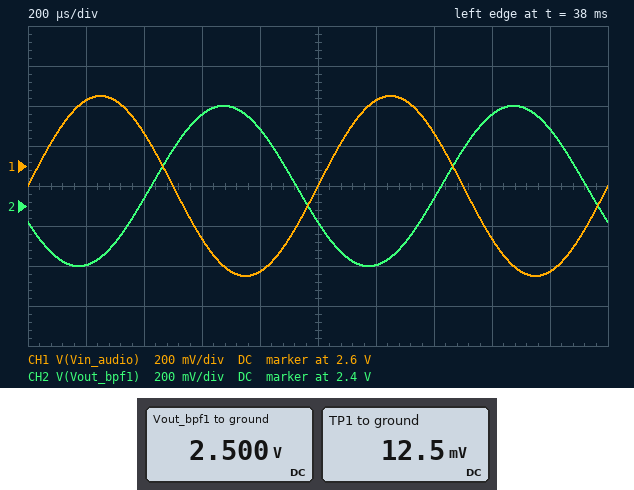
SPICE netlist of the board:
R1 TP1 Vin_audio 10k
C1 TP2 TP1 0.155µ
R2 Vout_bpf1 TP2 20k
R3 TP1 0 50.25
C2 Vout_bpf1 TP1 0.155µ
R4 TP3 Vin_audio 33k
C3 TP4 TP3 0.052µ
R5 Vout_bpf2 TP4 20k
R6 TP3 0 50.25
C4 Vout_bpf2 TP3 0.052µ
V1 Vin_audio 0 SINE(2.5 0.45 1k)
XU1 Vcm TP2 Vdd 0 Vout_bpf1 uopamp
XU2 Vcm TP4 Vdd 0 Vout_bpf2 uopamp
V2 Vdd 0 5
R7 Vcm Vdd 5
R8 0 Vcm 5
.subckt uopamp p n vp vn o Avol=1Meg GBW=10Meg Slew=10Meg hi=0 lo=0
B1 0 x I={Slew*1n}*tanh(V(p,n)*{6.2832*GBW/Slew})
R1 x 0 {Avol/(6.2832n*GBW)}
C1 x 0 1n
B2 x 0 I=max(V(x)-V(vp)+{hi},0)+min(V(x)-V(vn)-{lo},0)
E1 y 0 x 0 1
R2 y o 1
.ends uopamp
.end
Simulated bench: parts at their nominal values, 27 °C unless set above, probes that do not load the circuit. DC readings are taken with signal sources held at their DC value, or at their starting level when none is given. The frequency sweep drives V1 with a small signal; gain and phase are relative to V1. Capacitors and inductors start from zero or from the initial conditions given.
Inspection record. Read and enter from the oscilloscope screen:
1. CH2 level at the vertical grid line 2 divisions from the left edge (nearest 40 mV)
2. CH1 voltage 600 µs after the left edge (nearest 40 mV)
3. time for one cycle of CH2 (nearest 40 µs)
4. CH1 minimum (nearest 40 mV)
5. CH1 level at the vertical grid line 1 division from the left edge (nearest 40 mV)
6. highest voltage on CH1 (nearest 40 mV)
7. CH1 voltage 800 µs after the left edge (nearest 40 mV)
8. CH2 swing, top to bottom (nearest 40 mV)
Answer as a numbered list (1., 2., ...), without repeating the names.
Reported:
1. 2.44 V
2. 2.24 V
3. 1.00 ms
4. 2.04 V
5. 2.92 V
6. 2.96 V
7. 2.08 V
8. 800 mV
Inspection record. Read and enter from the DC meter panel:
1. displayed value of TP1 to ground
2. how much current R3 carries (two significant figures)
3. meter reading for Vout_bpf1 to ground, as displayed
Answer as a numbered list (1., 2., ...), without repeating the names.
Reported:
1. 12.5 mV
2. 250 µA
3. 2.500 V
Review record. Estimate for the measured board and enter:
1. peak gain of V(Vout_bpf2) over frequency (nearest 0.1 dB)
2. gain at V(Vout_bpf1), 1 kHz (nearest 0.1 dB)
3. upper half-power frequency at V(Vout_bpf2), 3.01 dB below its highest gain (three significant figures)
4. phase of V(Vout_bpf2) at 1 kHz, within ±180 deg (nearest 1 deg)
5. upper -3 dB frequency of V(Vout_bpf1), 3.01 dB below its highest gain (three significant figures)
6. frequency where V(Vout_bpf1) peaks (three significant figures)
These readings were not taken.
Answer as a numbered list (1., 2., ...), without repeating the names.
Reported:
1. -10.4 dB
2. -1.0 dB
3. 3.20 kHz
4. -92 deg
5. 1.08 kHz
6. 1.03 kHz
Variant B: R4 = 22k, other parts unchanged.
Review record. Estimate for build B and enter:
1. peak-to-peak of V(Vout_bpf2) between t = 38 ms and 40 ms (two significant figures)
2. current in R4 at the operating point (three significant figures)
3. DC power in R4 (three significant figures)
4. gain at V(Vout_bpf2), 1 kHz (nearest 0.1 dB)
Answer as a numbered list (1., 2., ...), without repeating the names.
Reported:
1. 15 mV
2. 113 µA
3. 283 µW
4. -35.6 dB
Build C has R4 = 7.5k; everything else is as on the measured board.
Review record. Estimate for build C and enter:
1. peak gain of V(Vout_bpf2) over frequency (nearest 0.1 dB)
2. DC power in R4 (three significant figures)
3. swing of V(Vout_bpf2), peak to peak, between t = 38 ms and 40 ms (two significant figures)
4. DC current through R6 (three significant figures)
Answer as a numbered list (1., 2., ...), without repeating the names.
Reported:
1. 2.5 dB
2. 822 µW
3. 44 mV
4. 331 µA
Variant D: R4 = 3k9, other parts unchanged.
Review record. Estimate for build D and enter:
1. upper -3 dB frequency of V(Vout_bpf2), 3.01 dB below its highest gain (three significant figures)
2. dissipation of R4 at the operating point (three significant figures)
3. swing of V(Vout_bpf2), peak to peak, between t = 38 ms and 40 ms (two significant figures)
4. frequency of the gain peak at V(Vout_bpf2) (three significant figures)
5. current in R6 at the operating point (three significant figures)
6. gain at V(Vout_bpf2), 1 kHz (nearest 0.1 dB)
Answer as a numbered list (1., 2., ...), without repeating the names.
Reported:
1. 3.22 kHz
2. 1.56 mW
3. 84 mV
4. 3.06 kHz
5. 633 µA
6. -20.6 dB
